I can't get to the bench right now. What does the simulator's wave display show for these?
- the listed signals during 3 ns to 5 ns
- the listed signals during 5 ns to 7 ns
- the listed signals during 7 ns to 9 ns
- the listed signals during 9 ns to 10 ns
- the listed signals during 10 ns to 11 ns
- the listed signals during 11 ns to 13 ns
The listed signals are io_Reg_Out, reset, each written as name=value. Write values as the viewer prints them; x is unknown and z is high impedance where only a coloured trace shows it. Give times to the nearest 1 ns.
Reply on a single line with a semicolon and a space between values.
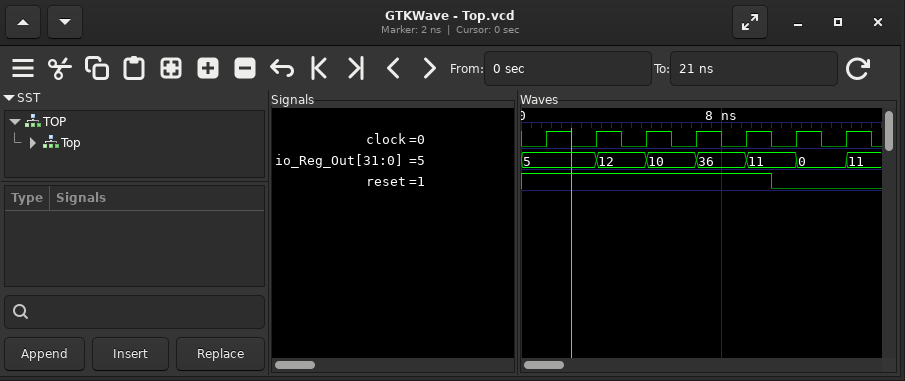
io_Reg_Out=12, reset=1; io_Reg_Out=10, reset=1; io_Reg_Out=36, reset=1; io_Reg_Out=11, reset=1; io_Reg_Out=11, reset=0; io_Reg_Out=0, reset=0
